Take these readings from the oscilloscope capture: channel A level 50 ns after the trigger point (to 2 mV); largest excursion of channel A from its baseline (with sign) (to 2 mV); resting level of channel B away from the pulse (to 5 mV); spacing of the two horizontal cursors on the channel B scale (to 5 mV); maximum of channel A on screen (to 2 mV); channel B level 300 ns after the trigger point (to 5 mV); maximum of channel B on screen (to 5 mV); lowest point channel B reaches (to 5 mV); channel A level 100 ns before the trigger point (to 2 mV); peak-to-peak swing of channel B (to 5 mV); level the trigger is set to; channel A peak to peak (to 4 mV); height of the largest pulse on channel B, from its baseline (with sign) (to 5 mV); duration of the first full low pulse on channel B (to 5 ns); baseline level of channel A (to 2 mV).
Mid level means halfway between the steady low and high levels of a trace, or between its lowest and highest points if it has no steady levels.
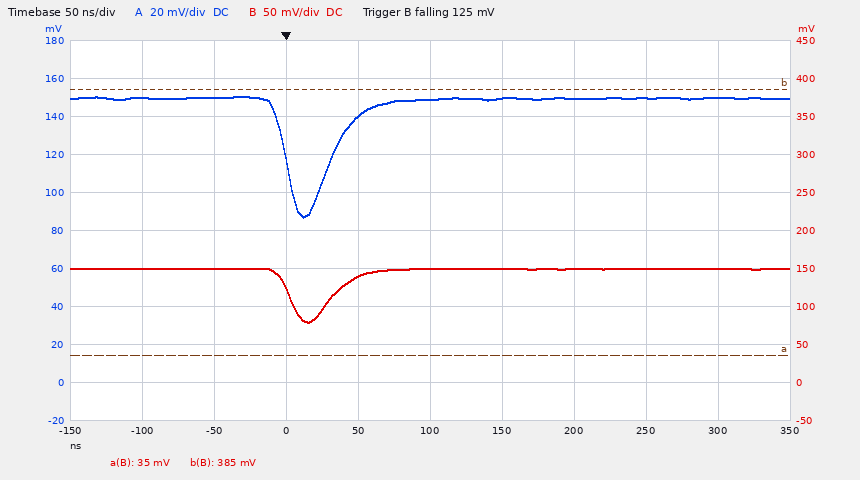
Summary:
140 mV
-62 mV
150 mV
350 mV
150 mV
150 mV
150 mV
80 mV
150 mV
70 mV
125 mV
64 mV
-70 mV
30 ns
150 mV
